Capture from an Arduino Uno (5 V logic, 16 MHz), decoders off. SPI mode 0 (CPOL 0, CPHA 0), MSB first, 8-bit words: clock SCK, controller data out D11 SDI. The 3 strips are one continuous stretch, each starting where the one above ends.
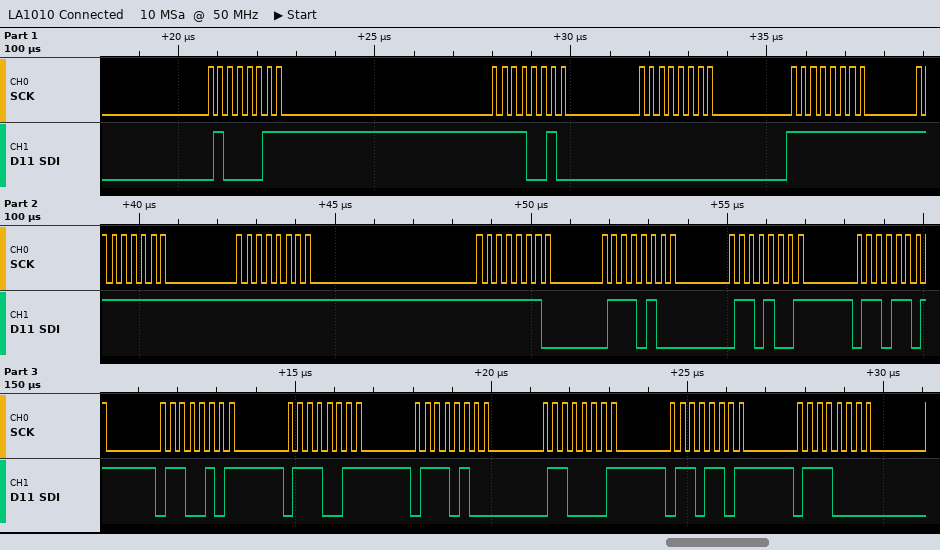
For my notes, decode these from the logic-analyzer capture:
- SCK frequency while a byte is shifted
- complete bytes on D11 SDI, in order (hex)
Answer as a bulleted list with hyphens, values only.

- 4 MHz
- 43 F2 00 FF FF FF FE 74 69 6D 65 73 74 61 6D 70
